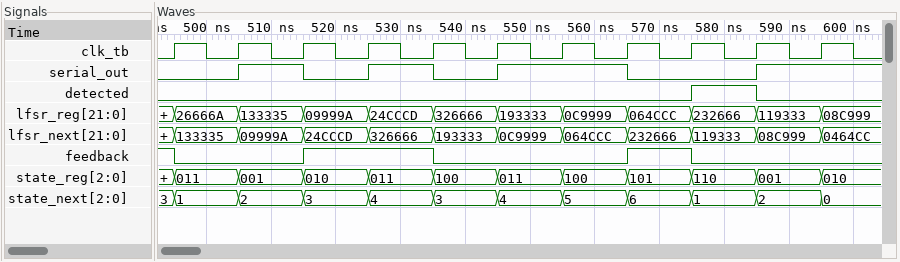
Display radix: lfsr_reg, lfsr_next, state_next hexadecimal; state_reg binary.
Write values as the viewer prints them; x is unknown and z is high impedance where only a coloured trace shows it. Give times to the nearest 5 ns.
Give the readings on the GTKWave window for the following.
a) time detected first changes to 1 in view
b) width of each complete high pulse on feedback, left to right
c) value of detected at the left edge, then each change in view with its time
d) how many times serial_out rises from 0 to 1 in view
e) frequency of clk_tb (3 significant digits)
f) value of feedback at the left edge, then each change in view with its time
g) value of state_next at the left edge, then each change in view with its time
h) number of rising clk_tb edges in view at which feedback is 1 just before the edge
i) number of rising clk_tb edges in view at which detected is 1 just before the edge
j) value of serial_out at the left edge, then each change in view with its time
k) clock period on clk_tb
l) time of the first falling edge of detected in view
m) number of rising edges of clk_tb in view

575 ns
20 ns, 10 ns
0, 1 at 575 ns, 0 at 585 ns
4
100 MHz
1, 0 at 495 ns, 1 at 515 ns, 0 at 535 ns, 1 at 565 ns, 0 at 575 ns
3, 1 at 495 ns, 2 at 505 ns, 3 at 515 ns, 4 at 525 ns, 3 at 535 ns, 4 at 545 ns, 5 at 555 ns, 6 at 565 ns, 1 at 575 ns, 2 at 585 ns, 0 at 595 ns
4
1
0, 1 at 505 ns, 0 at 515 ns, 1 at 525 ns, 0 at 535 ns, 1 at 545 ns, 0 at 565 ns, 1 at 585 ns
10 ns
585 ns
11
